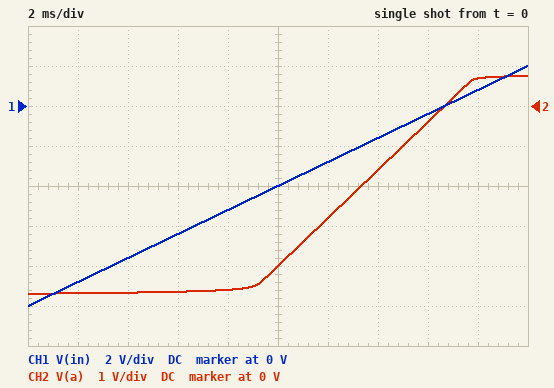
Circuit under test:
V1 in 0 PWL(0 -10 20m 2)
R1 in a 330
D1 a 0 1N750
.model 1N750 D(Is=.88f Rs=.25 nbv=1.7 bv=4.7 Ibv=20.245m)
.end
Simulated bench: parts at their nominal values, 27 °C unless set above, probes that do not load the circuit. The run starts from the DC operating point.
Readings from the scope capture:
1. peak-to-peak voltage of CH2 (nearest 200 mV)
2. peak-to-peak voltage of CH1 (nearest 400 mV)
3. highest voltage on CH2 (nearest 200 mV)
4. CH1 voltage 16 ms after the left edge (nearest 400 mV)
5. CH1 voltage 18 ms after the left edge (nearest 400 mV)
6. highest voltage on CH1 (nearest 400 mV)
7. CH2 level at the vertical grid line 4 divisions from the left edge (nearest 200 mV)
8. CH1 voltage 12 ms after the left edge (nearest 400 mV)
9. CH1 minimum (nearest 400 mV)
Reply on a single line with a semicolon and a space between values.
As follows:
5.4 V; 12.0 V; 800 mV; -400 mV; 800 mV; 2.0 V; -4.6 V; -2.8 V; -10.0 V
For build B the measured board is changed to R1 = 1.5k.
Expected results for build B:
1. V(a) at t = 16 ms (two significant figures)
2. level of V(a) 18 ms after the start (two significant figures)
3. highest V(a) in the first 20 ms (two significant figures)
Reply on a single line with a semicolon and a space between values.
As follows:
-400 mV; 660 mV; 710 mV
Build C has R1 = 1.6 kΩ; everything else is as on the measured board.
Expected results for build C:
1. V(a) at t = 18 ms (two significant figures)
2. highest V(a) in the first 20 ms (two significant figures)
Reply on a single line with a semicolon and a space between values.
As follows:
660 mV; 710 mV
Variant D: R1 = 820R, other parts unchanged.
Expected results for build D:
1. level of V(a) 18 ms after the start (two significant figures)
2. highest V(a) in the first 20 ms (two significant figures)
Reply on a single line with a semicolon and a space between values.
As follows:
670 mV; 730 mV
